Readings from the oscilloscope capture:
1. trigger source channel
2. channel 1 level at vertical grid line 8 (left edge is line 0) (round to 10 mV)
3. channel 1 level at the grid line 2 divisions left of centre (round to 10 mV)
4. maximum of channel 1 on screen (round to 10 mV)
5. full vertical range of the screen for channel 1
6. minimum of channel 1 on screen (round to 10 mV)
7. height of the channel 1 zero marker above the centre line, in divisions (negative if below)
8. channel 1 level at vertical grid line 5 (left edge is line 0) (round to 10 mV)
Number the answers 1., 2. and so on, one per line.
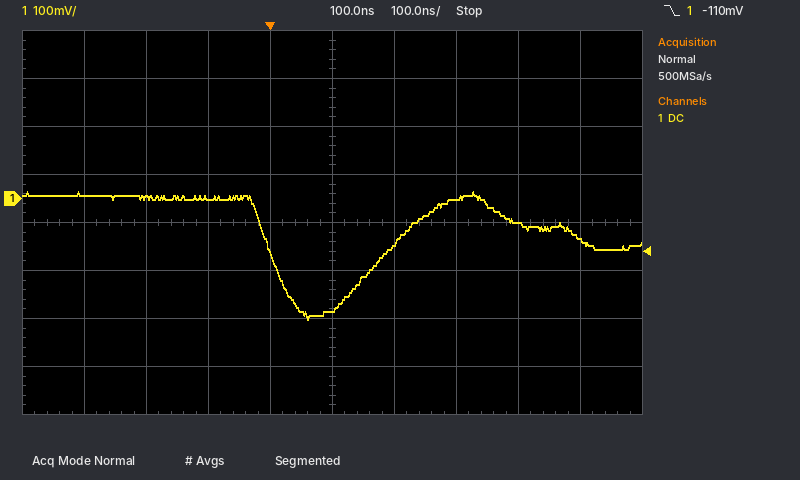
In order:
1. channel 1
2. -50 mV
3. 0 mV
4. 10 mV
5. 800 mV
6. -250 mV
7. +0.5 div
8. -230 mV
